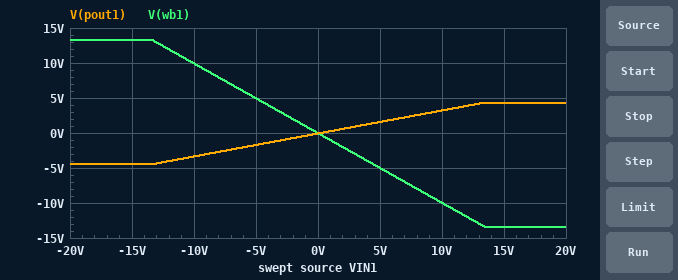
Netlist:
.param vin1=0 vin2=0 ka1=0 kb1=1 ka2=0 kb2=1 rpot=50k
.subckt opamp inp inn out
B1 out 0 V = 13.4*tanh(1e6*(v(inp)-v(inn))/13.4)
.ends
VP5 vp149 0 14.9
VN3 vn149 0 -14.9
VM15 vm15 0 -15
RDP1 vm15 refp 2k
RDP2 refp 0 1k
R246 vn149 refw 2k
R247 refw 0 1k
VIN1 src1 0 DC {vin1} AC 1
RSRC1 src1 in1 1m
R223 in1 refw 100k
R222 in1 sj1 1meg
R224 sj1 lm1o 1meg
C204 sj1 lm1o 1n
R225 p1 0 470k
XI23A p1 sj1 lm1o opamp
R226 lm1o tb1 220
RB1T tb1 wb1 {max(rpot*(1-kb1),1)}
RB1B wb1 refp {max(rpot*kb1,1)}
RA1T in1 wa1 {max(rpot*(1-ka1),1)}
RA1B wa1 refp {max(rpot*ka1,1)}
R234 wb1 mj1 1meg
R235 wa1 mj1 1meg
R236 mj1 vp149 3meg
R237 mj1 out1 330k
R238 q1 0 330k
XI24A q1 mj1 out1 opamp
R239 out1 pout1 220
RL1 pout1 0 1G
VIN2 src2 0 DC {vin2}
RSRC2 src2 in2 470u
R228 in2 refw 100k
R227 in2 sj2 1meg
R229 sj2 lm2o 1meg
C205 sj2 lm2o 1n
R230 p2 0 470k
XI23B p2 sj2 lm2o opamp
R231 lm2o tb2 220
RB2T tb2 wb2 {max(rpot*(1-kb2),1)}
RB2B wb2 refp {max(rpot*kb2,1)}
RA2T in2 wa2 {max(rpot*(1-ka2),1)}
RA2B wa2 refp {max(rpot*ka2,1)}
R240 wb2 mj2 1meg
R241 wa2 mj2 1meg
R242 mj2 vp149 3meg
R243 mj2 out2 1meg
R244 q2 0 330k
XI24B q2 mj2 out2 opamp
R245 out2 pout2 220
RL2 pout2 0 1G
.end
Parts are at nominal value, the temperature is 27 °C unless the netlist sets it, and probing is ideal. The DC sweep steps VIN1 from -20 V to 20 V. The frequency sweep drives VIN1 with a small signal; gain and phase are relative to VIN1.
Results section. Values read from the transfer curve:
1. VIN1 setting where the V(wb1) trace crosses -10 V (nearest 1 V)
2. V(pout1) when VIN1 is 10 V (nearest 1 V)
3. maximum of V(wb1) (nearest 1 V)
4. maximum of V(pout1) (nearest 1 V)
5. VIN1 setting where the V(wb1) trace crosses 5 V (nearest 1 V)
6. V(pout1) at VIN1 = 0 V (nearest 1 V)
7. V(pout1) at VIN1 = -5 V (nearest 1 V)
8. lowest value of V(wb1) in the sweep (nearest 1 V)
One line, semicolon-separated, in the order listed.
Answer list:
10 V; 3 V; 13 V; 4 V; -5 V; 0 V; -2 V; -13 V
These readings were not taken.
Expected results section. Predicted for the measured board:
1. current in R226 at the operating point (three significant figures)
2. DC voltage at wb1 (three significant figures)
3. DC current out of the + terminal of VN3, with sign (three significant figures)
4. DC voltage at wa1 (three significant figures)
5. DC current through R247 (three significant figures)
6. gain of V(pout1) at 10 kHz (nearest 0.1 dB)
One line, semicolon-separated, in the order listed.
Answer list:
94.4 µA; -20.9 mV; -5.00 mA; -4.74 V; 4.90 mA; -43.5 dB
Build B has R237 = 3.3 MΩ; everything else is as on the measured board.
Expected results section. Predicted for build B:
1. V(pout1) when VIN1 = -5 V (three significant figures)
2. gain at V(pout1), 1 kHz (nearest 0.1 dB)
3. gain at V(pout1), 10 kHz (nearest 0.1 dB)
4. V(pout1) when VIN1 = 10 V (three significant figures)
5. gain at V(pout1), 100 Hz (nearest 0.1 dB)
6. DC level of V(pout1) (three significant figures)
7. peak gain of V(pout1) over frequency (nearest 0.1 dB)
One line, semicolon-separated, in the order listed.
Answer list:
-13.4 V; -5.7 dB; -23.5 dB; 13.4 V; 8.9 dB; -675 mV; 10.3 dB
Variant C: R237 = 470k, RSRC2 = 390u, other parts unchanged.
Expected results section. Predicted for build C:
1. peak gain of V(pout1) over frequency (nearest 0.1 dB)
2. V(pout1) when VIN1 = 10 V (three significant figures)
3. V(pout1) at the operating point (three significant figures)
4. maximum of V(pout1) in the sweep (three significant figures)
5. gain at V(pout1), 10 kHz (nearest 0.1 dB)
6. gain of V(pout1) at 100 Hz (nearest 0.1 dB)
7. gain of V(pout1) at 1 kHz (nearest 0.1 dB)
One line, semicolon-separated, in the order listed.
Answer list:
-6.6 dB; 4.58 V; -96.1 mV; 6.17 V; -40.4 dB; -8.0 dB; -22.6 dB
